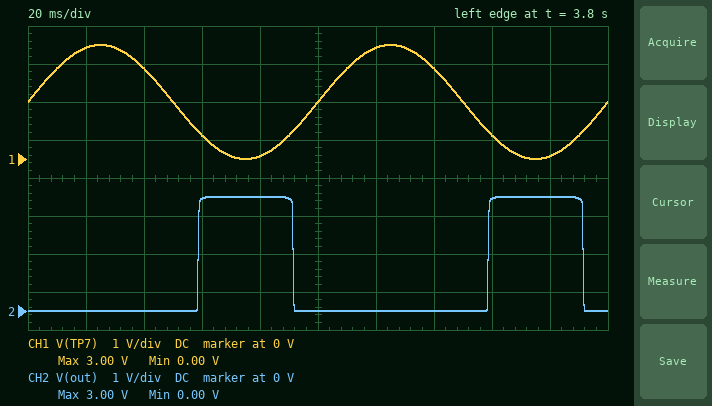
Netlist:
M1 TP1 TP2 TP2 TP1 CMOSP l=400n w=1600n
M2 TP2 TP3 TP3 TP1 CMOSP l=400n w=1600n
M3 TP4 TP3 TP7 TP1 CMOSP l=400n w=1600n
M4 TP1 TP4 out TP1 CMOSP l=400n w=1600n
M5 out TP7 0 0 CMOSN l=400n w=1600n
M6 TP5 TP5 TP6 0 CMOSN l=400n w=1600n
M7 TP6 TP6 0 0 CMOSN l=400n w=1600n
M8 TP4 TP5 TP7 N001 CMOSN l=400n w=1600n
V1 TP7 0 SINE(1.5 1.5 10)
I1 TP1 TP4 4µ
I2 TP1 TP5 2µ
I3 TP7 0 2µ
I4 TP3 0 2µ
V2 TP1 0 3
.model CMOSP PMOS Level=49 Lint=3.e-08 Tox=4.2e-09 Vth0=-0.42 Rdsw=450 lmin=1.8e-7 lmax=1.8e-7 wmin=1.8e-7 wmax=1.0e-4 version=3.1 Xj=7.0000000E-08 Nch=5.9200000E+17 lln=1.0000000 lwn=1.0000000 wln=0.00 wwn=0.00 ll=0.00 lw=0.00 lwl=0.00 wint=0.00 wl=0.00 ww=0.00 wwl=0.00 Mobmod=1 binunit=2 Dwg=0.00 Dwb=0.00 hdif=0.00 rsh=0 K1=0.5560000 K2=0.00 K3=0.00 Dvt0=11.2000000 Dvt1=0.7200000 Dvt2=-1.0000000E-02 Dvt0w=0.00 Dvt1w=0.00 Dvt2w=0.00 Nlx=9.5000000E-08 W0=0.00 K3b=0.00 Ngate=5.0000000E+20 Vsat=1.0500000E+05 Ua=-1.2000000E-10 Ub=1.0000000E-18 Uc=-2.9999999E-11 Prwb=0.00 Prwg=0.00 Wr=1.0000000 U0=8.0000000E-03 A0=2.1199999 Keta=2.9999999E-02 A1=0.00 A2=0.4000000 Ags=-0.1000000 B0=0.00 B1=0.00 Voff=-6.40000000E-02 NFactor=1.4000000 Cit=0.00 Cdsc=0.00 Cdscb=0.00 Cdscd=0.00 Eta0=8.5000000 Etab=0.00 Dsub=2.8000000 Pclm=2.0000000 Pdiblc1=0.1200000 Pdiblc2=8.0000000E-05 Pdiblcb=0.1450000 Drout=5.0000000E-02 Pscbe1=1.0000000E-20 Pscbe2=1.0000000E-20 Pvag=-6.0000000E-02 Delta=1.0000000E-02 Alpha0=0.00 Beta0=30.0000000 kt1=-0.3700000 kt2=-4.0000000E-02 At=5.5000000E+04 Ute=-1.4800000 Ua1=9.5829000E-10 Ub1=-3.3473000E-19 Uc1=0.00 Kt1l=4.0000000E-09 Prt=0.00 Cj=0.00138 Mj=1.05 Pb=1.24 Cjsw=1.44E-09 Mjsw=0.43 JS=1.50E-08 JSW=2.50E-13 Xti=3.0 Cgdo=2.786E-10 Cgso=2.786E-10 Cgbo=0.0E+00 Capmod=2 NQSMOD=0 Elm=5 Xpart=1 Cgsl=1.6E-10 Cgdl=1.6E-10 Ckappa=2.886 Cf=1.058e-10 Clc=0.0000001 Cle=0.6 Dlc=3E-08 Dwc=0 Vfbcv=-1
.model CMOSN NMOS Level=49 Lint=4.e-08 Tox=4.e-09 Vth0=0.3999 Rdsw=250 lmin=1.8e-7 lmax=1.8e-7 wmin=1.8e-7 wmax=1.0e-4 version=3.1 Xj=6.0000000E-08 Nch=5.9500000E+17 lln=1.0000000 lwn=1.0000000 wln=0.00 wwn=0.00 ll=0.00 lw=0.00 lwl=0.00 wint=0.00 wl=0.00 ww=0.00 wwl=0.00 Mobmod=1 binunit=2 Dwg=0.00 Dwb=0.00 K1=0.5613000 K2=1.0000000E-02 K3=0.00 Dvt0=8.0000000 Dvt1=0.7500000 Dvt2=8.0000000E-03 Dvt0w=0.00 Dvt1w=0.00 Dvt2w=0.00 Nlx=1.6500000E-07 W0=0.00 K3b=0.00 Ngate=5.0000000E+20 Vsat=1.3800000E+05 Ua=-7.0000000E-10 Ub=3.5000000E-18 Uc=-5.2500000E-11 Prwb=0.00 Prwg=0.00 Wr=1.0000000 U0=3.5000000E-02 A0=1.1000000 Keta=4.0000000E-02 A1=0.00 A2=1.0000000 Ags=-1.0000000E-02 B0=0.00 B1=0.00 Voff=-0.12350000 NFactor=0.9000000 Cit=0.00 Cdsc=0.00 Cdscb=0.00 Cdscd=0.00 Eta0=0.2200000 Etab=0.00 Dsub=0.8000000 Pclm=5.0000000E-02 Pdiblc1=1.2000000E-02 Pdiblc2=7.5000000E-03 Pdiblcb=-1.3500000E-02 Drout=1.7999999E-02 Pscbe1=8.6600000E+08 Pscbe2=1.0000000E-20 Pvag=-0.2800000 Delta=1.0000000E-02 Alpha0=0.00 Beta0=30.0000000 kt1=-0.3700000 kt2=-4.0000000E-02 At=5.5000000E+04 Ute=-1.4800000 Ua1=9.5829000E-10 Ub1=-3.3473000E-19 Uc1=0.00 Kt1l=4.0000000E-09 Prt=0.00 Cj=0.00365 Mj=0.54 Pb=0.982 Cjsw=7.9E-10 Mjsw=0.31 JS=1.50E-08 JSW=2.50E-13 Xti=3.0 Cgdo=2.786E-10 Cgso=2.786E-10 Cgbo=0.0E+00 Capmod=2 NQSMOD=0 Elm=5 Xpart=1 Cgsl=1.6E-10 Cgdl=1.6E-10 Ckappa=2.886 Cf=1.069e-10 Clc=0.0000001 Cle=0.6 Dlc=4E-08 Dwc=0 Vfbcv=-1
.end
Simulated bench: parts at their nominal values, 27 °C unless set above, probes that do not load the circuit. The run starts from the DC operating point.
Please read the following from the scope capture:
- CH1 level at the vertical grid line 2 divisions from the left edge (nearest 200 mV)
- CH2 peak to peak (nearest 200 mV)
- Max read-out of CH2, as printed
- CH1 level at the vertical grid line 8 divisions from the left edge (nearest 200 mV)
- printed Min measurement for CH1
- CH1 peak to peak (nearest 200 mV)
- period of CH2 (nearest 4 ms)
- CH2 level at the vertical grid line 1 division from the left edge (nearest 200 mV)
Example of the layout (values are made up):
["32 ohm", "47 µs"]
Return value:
["2.4 V", "3.0 V", "3.00 V", "600 mV", "0.00 V", "3.0 V", "100 ms", "0 V"]
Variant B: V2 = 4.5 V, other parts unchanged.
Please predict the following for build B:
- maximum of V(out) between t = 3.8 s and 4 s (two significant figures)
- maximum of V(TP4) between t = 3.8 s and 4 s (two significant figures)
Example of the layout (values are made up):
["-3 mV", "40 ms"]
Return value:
["4.5 V", "3.9 V"]
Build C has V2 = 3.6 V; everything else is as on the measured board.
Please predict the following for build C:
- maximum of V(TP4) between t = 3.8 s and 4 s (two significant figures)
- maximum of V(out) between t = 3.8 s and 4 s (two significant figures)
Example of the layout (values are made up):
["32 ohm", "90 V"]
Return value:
["3.1 V", "3.6 V"]
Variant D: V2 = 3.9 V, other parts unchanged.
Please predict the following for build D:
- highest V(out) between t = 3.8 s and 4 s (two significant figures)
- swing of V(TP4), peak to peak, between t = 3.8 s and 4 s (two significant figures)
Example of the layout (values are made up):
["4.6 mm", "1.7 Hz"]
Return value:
["3.9 V", "3.3 V"]
